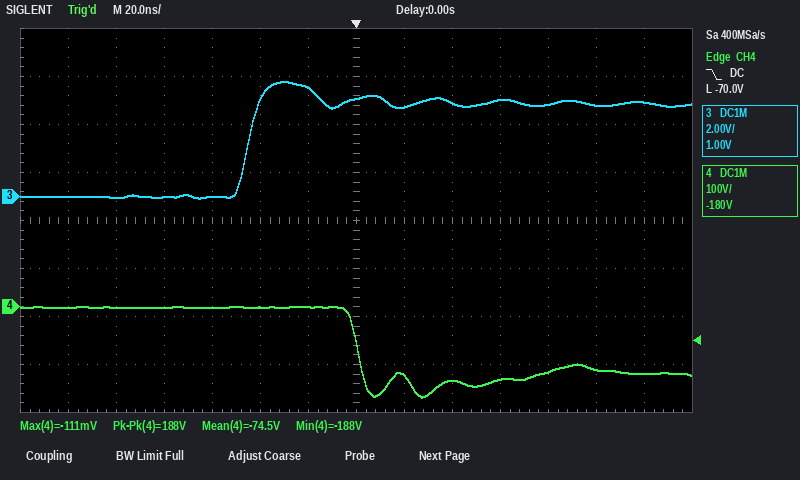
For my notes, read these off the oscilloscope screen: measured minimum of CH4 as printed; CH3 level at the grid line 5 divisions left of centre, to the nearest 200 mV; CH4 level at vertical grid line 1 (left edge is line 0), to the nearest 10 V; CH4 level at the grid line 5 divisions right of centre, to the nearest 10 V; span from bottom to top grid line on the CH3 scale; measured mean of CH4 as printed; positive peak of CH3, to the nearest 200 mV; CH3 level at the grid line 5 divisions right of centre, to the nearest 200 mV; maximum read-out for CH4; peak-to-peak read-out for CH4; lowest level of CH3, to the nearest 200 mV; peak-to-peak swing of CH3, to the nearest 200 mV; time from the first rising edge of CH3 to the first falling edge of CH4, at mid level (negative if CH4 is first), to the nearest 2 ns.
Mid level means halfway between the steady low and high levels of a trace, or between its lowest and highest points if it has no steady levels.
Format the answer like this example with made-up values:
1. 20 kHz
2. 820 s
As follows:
1. -188 V
2. 0.0 V
3. 0 V
4. -130 V
5. 16 V
6. -74.5 V
7. 4.8 V
8. 3.8 V
9. -111 mV
10. 188 V
11. 0.0 V
12. 4.8 V
13. +46 ns
